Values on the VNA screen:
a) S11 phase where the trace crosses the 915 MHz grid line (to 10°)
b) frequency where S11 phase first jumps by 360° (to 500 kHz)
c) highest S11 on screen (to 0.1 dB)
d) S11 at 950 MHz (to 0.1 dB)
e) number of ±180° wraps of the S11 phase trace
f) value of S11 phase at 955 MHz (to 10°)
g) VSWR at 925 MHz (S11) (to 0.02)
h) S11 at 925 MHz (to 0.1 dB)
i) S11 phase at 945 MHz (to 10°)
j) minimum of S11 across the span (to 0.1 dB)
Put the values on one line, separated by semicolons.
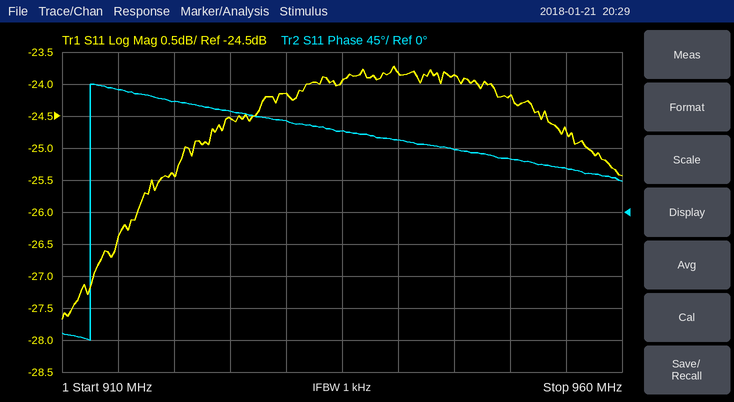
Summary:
170°; 912.5 MHz; -23.7 dB; -24.2 dB; 1; 60°; 1.12; -24.5 dB; 90°; -27.7 dB
